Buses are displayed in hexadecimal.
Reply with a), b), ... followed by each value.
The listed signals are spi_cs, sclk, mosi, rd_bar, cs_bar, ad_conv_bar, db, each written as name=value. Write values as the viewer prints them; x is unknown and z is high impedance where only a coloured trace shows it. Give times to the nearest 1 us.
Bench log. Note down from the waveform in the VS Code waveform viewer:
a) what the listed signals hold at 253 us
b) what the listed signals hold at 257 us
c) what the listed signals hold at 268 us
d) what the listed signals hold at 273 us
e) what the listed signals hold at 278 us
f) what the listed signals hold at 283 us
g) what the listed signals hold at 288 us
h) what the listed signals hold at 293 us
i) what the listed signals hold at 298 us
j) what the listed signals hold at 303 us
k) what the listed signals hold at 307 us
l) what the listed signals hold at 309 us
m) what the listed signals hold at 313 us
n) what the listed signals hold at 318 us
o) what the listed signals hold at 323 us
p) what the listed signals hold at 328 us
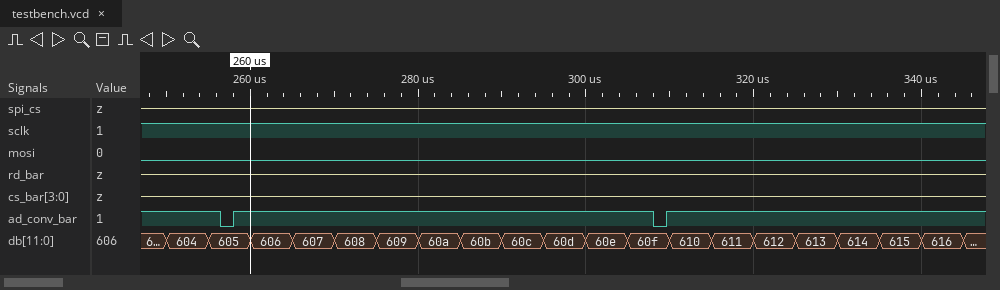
a) spi_cs=z, sclk=1, mosi=0, rd_bar=z, cs_bar=z, ad_conv_bar=1, db=604
b) spi_cs=z, sclk=1, mosi=0, rd_bar=z, cs_bar=z, ad_conv_bar=0, db=605
c) spi_cs=z, sclk=1, mosi=0, rd_bar=z, cs_bar=z, ad_conv_bar=1, db=607
d) spi_cs=z, sclk=1, mosi=0, rd_bar=z, cs_bar=z, ad_conv_bar=1, db=608
e) spi_cs=z, sclk=1, mosi=0, rd_bar=z, cs_bar=z, ad_conv_bar=1, db=609
f) spi_cs=z, sclk=1, mosi=0, rd_bar=z, cs_bar=z, ad_conv_bar=1, db=60a
g) spi_cs=z, sclk=1, mosi=0, rd_bar=z, cs_bar=z, ad_conv_bar=1, db=60b
h) spi_cs=z, sclk=1, mosi=0, rd_bar=z, cs_bar=z, ad_conv_bar=1, db=60c
i) spi_cs=z, sclk=1, mosi=0, rd_bar=z, cs_bar=z, ad_conv_bar=1, db=60d
j) spi_cs=z, sclk=1, mosi=0, rd_bar=z, cs_bar=z, ad_conv_bar=1, db=60e
k) spi_cs=z, sclk=1, mosi=0, rd_bar=z, cs_bar=z, ad_conv_bar=1, db=60f
l) spi_cs=z, sclk=1, mosi=0, rd_bar=z, cs_bar=z, ad_conv_bar=0, db=60f
m) spi_cs=z, sclk=1, mosi=0, rd_bar=z, cs_bar=z, ad_conv_bar=1, db=610
n) spi_cs=z, sclk=1, mosi=0, rd_bar=z, cs_bar=z, ad_conv_bar=1, db=611
o) spi_cs=z, sclk=1, mosi=0, rd_bar=z, cs_bar=z, ad_conv_bar=1, db=612
p) spi_cs=z, sclk=1, mosi=0, rd_bar=z, cs_bar=z, ad_conv_bar=1, db=613
